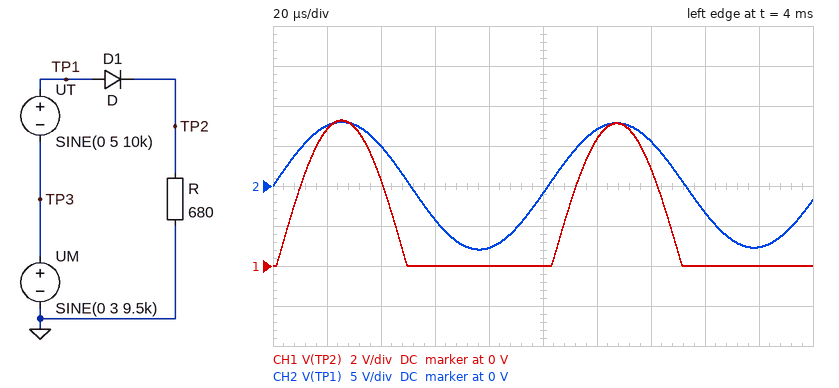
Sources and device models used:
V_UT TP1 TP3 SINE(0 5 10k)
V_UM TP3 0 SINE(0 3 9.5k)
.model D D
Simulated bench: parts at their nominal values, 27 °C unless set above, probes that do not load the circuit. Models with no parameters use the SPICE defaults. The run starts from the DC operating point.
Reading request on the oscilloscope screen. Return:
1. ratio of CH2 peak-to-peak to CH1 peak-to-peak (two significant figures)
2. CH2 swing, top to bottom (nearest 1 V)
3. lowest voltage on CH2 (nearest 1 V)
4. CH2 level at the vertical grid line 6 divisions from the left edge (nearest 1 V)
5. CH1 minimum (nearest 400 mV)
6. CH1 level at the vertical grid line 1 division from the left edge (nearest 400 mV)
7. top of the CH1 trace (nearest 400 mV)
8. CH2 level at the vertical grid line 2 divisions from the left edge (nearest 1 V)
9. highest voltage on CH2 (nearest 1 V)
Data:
2.2
16 V
-8 V
7 V
0 V
6.8 V
7.2 V
5 V
8 V
